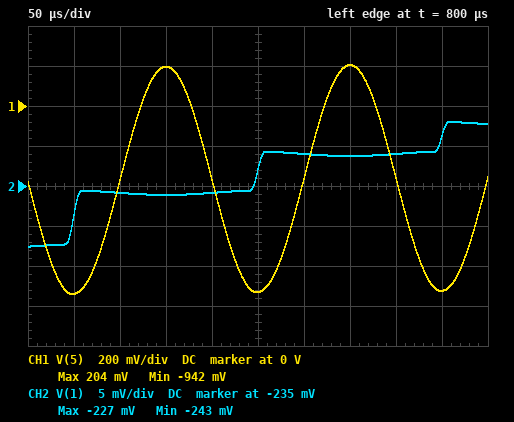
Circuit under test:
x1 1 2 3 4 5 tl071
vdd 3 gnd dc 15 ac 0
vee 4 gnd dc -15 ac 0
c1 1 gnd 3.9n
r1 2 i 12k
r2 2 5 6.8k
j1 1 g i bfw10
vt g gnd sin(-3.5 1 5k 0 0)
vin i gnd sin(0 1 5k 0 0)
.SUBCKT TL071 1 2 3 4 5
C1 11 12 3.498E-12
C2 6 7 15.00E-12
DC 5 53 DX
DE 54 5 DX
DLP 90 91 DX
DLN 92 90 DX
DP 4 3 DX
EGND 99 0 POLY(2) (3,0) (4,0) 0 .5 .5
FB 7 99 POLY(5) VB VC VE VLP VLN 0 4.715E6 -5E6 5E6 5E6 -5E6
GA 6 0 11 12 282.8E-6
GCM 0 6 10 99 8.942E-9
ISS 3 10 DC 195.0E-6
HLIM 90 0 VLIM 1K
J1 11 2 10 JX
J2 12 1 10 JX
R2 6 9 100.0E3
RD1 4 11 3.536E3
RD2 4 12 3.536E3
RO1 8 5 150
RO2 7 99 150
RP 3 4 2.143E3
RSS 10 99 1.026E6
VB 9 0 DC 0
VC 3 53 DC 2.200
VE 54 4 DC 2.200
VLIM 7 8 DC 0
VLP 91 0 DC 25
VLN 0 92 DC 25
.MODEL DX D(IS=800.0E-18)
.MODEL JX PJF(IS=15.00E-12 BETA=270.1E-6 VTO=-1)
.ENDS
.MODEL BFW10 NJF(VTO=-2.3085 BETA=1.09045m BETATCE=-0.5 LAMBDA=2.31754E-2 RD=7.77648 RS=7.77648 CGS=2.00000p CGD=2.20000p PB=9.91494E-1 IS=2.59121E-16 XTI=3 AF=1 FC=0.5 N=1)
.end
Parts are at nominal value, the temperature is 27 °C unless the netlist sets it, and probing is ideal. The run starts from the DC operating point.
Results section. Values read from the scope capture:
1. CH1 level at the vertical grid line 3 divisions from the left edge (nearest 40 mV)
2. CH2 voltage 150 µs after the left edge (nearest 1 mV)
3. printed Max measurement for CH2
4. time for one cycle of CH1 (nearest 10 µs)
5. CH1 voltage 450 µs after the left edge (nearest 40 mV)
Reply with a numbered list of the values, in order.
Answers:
1. 200 mV
2. -236 mV
3. -227 mV
4. 200 µs
5. -920 mV
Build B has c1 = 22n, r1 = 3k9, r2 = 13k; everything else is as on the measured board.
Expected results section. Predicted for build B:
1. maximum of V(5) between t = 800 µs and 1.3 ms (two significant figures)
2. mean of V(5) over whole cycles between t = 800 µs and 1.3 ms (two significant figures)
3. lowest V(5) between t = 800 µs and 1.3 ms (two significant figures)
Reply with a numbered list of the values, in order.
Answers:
1. 2.0 V
2. -1.4 V
3. -4.8 V
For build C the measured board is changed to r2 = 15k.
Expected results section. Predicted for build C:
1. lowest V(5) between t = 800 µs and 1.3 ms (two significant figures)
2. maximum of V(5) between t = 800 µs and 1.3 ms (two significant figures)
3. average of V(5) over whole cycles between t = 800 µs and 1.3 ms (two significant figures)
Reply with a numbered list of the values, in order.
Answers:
1. -1.8 V
2. 730 mV
3. -530 mV
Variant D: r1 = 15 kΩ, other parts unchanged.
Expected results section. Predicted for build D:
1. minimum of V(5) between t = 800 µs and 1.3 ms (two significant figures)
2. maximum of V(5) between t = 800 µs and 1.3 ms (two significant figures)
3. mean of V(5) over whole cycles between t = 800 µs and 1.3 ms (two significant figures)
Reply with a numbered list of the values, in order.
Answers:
1. -800 mV
2. 120 mV
3. -340 mV
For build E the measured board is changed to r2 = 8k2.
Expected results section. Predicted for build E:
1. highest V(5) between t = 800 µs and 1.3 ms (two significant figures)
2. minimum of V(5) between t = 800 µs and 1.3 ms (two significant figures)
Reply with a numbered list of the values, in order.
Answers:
1. 290 mV
2. -1.1 V
